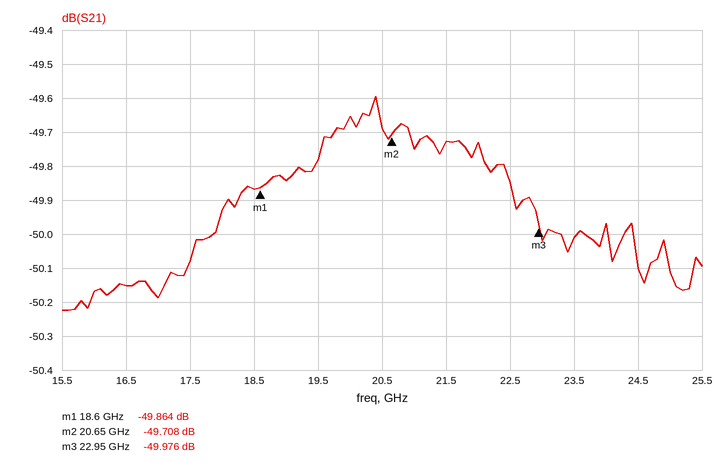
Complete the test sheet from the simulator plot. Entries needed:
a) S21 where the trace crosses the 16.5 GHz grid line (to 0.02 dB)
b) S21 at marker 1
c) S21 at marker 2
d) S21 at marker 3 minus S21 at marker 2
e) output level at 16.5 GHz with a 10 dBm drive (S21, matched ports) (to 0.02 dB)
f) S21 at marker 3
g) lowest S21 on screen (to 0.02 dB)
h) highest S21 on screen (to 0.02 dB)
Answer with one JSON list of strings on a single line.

["-50.16 dB", "-49.864 dB", "-49.708 dB", "-0.268 dB", "-40.16 dBm", "-49.976 dB", "-50.22 dB", "-49.60 dB"]
